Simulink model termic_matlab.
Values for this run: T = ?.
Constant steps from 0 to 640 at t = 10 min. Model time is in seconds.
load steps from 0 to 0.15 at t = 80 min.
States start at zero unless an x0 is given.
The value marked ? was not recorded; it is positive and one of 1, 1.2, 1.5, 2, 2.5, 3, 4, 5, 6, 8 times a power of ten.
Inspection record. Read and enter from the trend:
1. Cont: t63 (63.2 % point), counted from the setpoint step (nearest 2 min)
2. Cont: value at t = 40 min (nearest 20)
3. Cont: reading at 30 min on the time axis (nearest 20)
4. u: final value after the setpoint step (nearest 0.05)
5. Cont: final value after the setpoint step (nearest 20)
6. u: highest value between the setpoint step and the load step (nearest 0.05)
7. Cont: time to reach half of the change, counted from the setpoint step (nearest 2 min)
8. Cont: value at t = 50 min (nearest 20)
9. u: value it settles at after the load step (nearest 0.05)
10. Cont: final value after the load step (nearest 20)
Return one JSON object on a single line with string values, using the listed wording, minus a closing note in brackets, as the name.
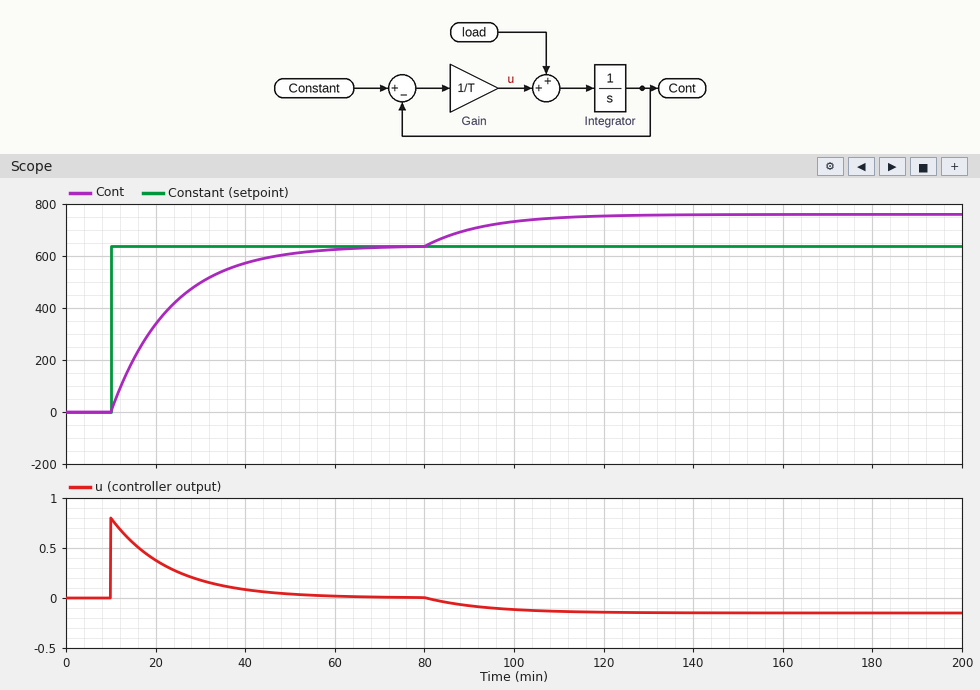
{"Cont: t63 (63.2 % point), counted from the setpoint step": "14 min", "Cont: value at t = 40 min": "580", "Cont: reading at 30 min on the time axis": "500", "u: final value after the setpoint step": "0.00", "Cont: final value after the setpoint step": "640", "u: highest value between the setpoint step and the load step": "0.80", "Cont: time to reach half of the change, counted from the setpoint step": "10 min", "Cont: value at t = 50 min": "600", "u: value it settles at after the load step": "-0.15", "Cont: final value after the load step": "760"}
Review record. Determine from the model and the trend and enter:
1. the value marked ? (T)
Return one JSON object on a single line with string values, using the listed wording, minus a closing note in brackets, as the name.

{"the value marked ?": "800"}
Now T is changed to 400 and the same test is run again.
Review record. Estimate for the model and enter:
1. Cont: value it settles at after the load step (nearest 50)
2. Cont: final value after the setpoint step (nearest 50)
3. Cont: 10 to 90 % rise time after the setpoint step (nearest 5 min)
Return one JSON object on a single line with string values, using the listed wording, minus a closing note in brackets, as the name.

{"Cont: value it settles at after the load step": "700", "Cont: final value after the setpoint step": "650", "Cont: 10 to 90 % rise time after the setpoint step": "15 min"}
